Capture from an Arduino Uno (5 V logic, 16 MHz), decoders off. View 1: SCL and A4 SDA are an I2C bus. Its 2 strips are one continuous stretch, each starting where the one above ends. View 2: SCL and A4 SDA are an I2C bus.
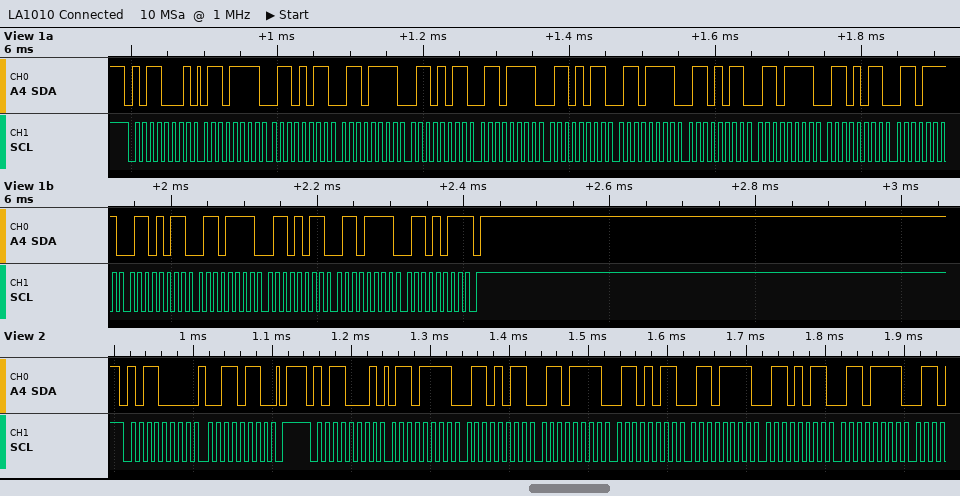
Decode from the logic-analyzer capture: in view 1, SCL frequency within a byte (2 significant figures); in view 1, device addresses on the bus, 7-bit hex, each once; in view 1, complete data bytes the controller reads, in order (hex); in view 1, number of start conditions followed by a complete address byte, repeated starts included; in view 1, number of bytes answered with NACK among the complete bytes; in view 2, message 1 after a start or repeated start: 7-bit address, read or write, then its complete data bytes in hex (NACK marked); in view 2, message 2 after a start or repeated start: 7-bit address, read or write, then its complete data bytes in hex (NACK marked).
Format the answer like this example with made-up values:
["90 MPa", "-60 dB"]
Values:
["100 kHz", "0x58", "6F 6B 6F 6B 6F 6B 6F 6B 6F 6B 6F 6B 6F 6B 6F 6B", "1", "1", "0x58 write: 36", "0x58 read: 6F 6B 6F 6B 6F 6B 6F"]
